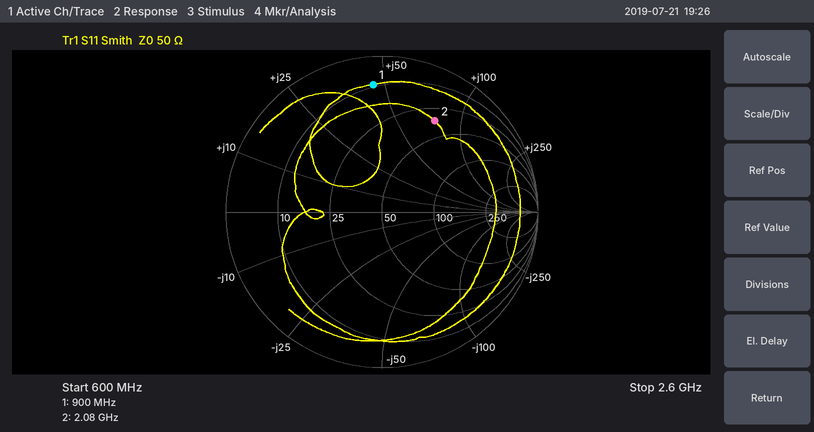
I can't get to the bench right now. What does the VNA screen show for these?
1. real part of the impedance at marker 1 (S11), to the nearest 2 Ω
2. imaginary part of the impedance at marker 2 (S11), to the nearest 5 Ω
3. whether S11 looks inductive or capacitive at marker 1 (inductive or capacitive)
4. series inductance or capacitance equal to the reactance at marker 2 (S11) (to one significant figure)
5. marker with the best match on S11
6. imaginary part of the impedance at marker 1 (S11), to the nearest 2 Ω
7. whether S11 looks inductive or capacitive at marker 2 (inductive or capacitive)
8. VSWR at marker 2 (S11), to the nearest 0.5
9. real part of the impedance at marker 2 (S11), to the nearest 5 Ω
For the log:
10 Ω
+75 Ω
inductive
6 nH
marker 2
+46 Ω
inductive
5.0
35 Ω
